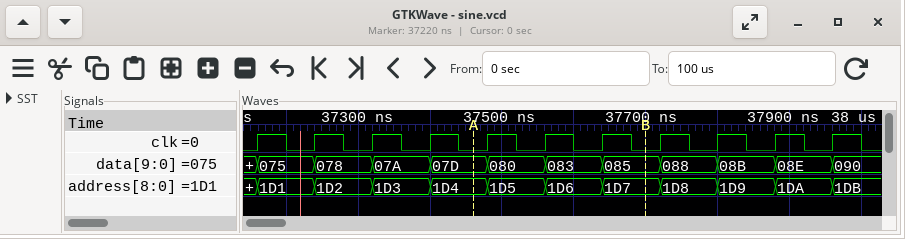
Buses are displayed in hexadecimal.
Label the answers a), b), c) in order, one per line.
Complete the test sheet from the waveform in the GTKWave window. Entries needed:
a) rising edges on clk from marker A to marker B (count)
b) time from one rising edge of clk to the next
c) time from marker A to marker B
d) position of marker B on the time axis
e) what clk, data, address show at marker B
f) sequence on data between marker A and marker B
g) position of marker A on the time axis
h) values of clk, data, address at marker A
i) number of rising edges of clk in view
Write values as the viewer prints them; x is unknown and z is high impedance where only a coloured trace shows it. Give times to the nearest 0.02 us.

a) 3
b) 0.08 us
c) 0.24 us
d) 37.7 us
e) clk=0, data=085, address=1D7
f) 07D, 080, 083, 085
g) 37.46 us
h) clk=0, data=07D, address=1D4
i) 11
